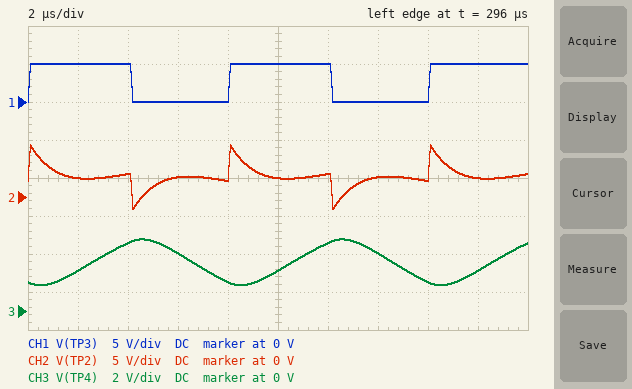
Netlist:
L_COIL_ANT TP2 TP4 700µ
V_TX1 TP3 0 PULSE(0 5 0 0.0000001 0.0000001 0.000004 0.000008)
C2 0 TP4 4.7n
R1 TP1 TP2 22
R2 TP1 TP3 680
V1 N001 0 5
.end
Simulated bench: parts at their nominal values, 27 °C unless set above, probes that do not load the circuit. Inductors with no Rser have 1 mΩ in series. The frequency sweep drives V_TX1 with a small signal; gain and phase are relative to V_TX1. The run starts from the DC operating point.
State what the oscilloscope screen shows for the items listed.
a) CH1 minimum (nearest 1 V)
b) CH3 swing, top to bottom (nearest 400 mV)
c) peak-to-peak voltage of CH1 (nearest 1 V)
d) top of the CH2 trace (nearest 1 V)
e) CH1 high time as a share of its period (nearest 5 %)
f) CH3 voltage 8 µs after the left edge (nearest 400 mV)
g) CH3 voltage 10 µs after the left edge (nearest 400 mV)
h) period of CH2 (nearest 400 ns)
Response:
0 V
2.4 V
5 V
7 V
50 %
1.6 V
2.0 V
8.0 µs
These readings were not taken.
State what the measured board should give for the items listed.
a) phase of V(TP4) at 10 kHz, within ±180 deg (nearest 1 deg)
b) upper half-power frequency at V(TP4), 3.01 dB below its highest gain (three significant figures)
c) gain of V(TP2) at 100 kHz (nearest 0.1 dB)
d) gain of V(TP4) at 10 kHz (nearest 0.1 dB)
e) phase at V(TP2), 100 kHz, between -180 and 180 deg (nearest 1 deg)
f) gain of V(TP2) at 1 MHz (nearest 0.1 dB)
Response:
-12 deg
64.5 kHz
-16.9 dB
-0.1 dB
82 deg
-0.1 dB
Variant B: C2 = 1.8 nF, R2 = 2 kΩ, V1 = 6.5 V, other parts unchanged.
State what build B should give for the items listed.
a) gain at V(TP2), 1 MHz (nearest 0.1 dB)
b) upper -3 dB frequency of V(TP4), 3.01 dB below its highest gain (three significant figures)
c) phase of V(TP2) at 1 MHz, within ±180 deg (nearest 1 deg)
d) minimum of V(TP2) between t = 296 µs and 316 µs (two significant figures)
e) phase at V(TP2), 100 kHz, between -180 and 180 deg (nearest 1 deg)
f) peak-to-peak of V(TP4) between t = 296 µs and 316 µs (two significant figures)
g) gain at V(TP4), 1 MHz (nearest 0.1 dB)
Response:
-0.9 dB
48.3 kHz
25 deg
-700 mV
-78 deg
2.5 V
-34.6 dB
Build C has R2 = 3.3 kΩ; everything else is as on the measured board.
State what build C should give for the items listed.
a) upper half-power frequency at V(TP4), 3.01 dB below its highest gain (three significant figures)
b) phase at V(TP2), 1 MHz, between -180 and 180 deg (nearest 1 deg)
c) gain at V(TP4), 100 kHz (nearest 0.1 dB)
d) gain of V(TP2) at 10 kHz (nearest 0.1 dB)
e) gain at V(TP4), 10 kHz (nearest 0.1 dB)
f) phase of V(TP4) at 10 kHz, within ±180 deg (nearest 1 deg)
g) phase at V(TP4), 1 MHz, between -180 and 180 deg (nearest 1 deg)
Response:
10.3 kHz
37 deg
-19.8 dB
-3.0 dB
-2.9 dB
-45 deg
-143 deg
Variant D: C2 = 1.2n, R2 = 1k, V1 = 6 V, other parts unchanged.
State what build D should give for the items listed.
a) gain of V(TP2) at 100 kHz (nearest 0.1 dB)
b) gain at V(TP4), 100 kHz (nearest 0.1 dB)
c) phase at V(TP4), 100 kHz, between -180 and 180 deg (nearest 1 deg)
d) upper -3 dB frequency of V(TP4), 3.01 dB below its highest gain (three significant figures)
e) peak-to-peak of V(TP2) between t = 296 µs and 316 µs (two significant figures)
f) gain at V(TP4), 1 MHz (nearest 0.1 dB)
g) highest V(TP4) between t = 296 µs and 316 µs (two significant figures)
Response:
-3.7 dB
-0.2 dB
-49 deg
182 kHz
5.1 V
-30.4 dB
5.3 V
